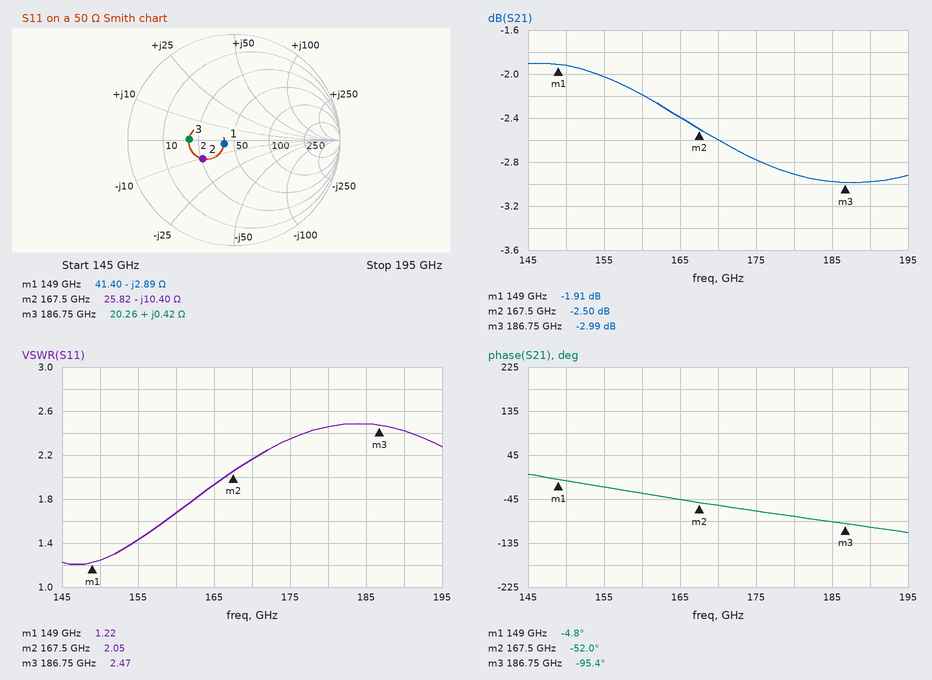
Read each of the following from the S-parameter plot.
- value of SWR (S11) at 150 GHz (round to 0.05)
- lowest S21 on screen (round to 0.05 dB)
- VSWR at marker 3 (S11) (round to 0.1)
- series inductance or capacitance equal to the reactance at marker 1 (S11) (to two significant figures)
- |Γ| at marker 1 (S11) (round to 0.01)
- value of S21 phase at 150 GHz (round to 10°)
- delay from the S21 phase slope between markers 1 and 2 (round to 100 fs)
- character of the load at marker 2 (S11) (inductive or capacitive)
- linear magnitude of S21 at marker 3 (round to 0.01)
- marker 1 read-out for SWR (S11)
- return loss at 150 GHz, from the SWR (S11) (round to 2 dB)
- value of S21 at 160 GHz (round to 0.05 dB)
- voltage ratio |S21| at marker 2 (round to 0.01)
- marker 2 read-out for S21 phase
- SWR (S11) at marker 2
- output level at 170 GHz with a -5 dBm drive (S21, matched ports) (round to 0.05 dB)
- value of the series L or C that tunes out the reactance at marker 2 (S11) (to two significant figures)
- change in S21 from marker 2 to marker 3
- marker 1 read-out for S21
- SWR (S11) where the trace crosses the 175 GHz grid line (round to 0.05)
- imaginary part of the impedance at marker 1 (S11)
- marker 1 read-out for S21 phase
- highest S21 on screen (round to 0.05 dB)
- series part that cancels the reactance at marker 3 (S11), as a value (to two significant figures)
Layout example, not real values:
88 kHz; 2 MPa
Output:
1.25; -3.00 dB; 2.5; 370 fF; 0.10; -10°; 7.1 ps; capacitive; 0.71; 1.22; 20 dB; -2.20 dB; 0.75; -52.0°; 2.05; -7.60 dBm; 9.9 pH; -0.49 dB; -1.91 dB; 2.35; -2.89 Ω; -4.8°; -1.90 dB; 2.0 pF
